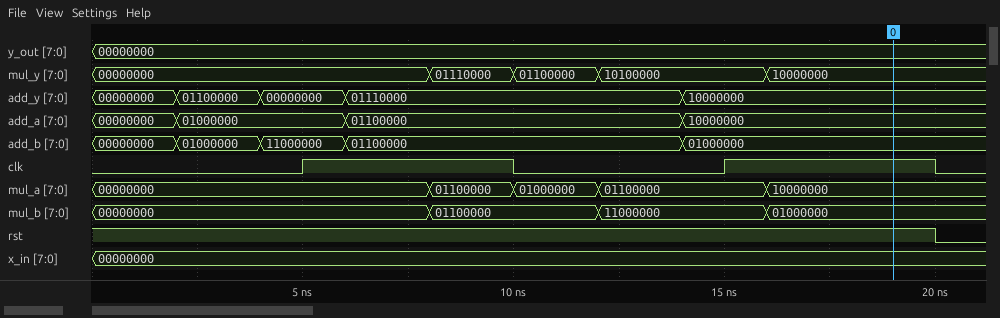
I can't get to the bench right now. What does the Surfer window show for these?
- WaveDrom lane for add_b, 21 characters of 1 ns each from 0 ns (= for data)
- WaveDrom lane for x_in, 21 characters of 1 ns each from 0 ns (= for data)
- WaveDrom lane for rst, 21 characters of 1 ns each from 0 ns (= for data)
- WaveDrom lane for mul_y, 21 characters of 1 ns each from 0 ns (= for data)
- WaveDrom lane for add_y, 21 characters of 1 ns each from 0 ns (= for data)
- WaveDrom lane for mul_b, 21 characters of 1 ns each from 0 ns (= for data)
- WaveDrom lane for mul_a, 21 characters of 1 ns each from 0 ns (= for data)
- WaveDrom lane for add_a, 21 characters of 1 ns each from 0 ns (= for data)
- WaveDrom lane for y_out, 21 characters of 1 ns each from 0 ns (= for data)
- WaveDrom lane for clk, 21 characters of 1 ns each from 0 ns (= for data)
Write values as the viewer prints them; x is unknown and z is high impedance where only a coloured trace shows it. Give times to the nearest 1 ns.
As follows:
{name: 'add_b', wave: '=.=.=.=.......=......', data: '00000000 01000000 11000000 01100000 01000000'}
{name: 'x_in', wave: '=....................', data: '00000000'}
{name: 'rst', wave: '1...................0'}
{name: 'mul_y', wave: '=.......=.=.=...=....', data: '00000000 01110000 01100000 10100000 10000000'}
{name: 'add_y', wave: '=.=.=.=.......=......', data: '00000000 01100000 00000000 01110000 10000000'}
{name: 'mul_b', wave: '=.......=...=...=....', data: '00000000 01100000 11000000 01000000'}
{name: 'mul_a', wave: '=.......=.=.=...=....', data: '00000000 01100000 01000000 01100000 10000000'}
{name: 'add_a', wave: '=.=...=.......=......', data: '00000000 01000000 01100000 10000000'}
{name: 'y_out', wave: '=....................', data: '00000000'}
{name: 'clk', wave: '0....1....0....1....0'}
